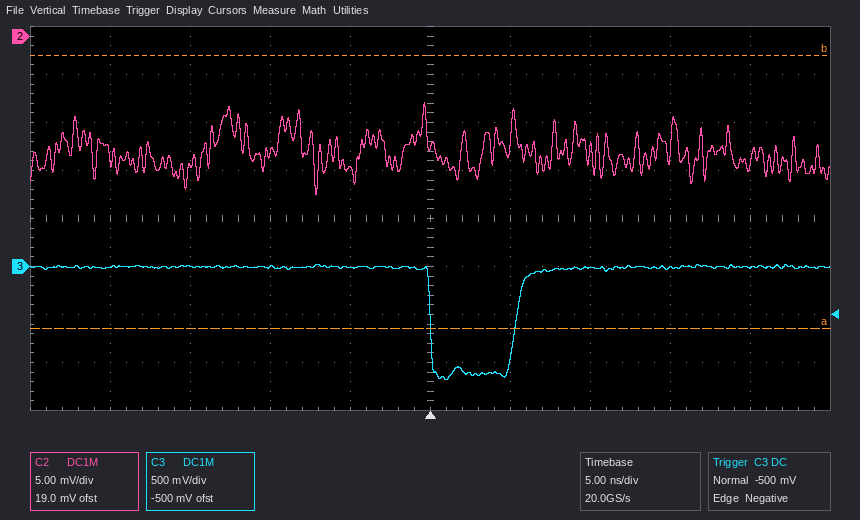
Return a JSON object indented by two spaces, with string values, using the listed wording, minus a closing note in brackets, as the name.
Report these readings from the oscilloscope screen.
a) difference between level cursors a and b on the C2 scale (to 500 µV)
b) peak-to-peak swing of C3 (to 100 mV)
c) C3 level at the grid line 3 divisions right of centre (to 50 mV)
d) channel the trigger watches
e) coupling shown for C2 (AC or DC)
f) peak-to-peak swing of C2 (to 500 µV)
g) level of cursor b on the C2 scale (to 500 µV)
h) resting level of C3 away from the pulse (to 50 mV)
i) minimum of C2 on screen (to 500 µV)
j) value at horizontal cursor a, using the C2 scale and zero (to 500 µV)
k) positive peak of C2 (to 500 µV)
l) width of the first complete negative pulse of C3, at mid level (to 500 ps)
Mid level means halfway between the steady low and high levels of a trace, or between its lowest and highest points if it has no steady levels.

{
  "difference between level cursors a and b on the C2 scale": "28.5 mV",
  "peak-to-peak swing of C3": "1.20 V",
  "C3 level at the grid line 3 divisions right of centre": "0 mV",
  "channel the trigger watches": "C3",
  "coupling shown for C2": "DC",
  "peak-to-peak swing of C2": "9.5 mV",
  "level of cursor b on the C2 scale": "-2.0 mV",
  "resting level of C3 away from the pulse": "0 mV",
  "minimum of C2 on screen": "-16.5 mV",
  "value at horizontal cursor a, using the C2 scale and zero": "-30.5 mV",
  "positive peak of C2": "-7.0 mV",
  "width of the first complete negative pulse of C3, at mid level": "5.5 ns"
}
